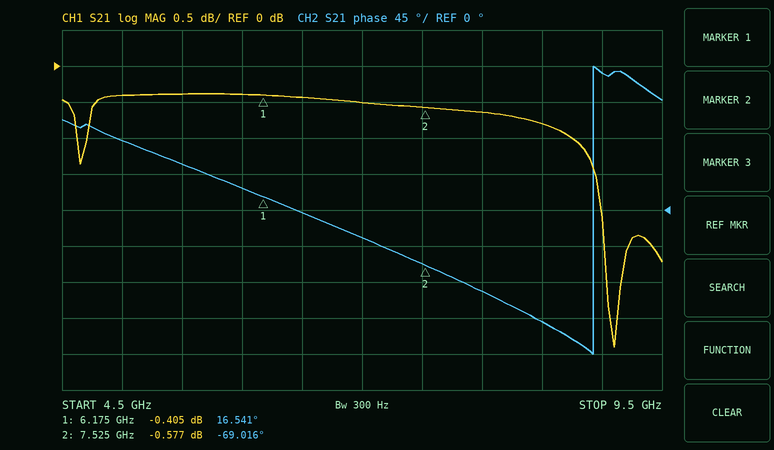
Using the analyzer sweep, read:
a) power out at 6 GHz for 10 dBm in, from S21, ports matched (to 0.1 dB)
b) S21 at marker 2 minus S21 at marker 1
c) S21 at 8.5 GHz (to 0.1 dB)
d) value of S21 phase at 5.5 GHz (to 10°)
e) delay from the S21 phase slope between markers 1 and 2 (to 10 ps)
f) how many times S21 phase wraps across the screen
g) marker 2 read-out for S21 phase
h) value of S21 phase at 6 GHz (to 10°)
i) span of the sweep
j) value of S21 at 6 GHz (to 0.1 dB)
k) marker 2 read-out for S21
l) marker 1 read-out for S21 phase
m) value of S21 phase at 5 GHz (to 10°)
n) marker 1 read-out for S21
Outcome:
9.6 dBm
-0.172 dB
-0.8 dB
60°
180 ps
1
-69.016°
30°
5 GHz
-0.4 dB
-0.577 dB
16.541°
90°
-0.405 dB
